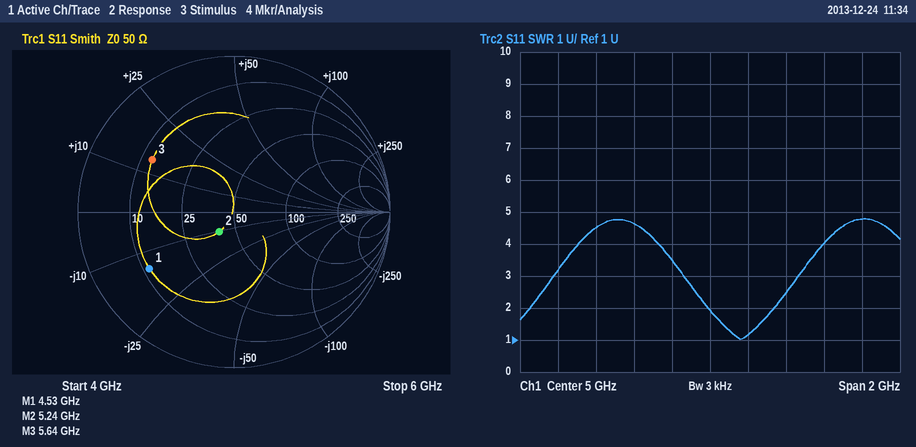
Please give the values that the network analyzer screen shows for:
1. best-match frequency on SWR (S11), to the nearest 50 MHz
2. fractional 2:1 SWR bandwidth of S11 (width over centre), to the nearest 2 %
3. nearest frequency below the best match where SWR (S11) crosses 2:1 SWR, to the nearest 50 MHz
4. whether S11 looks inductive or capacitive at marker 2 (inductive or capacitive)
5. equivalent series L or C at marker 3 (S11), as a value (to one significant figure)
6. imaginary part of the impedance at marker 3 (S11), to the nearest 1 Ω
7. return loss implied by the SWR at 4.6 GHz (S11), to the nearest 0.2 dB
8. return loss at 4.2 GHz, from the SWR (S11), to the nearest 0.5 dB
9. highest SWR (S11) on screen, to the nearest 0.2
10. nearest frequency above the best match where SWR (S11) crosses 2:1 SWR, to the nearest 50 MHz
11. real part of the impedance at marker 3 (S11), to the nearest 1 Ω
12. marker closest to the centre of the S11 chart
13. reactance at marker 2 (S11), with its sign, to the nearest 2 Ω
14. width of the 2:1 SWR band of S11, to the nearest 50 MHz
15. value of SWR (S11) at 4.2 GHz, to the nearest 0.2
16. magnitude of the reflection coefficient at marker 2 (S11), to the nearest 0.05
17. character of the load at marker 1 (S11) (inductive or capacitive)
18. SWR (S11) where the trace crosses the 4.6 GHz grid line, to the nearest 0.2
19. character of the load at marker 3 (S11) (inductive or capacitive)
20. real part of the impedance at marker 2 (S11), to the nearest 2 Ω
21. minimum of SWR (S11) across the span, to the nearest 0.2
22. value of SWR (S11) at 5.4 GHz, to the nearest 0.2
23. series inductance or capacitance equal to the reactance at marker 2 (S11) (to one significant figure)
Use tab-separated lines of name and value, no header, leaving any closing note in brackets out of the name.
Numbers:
best-match frequency on SWR (S11), to the nearest 50 MHz	5.15 GHz
fractional 2:1 SWR bandwidth of S11 (width over centre), to the nearest 2 %	6 %
nearest frequency below the best match where SWR (S11) crosses 2:1 SWR, to the nearest 50 MHz	5.00 GHz
whether S11 looks inductive or capacitive at marker 2	capacitive
equivalent series L or C at marker 3 (S11), as a value	400 pH
imaginary part of the impedance at marker 3 (S11), to the nearest 1 Ω	+14 Ω
return loss implied by the SWR at 4.6 GHz (S11), to the nearest 0.2 dB	3.8 dB
return loss at 4.2 GHz, from the SWR (S11), to the nearest 0.5 dB	5.5 dB
highest SWR (S11) on screen, to the nearest 0.2	4.8
nearest frequency above the best match where SWR (S11) crosses 2:1 SWR, to the nearest 50 MHz	5.35 GHz
real part of the impedance at marker 3 (S11), to the nearest 1 Ω	13 Ω
marker closest to the centre of the S11 chart	marker 2
reactance at marker 2 (S11), with its sign, to the nearest 2 Ω	-10 Ω
width of the 2:1 SWR band of S11, to the nearest 50 MHz	350 MHz
value of SWR (S11) at 4.2 GHz, to the nearest 0.2	3.2
magnitude of the reflection coefficient at marker 2 (S11), to the nearest 0.05	0.15
character of the load at marker 1 (S11)	capacitive
SWR (S11) where the trace crosses the 4.6 GHz grid line, to the nearest 0.2	4.6
character of the load at marker 3 (S11)	inductive
real part of the impedance at marker 2 (S11), to the nearest 2 Ω	40 Ω
minimum of SWR (S11) across the span, to the nearest 0.2	1.0
value of SWR (S11) at 5.4 GHz, to the nearest 0.2	2.4
series inductance or capacitance equal to the reactance at marker 2 (S11)	3 pF
